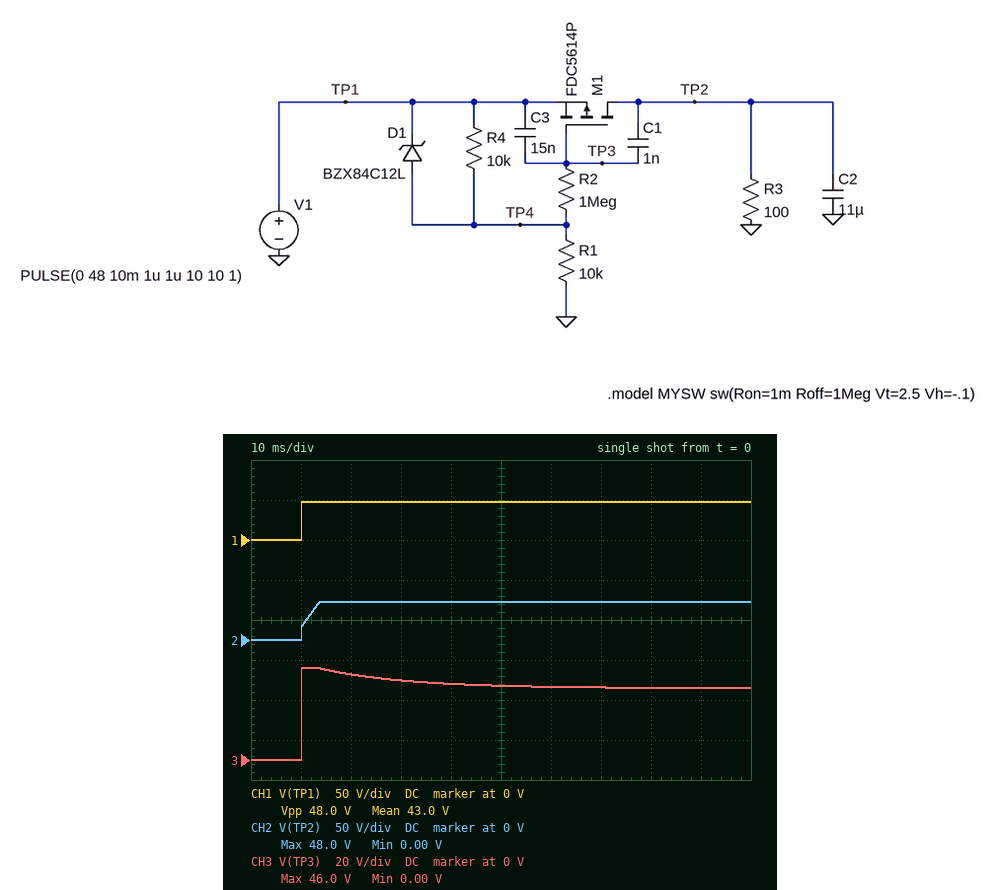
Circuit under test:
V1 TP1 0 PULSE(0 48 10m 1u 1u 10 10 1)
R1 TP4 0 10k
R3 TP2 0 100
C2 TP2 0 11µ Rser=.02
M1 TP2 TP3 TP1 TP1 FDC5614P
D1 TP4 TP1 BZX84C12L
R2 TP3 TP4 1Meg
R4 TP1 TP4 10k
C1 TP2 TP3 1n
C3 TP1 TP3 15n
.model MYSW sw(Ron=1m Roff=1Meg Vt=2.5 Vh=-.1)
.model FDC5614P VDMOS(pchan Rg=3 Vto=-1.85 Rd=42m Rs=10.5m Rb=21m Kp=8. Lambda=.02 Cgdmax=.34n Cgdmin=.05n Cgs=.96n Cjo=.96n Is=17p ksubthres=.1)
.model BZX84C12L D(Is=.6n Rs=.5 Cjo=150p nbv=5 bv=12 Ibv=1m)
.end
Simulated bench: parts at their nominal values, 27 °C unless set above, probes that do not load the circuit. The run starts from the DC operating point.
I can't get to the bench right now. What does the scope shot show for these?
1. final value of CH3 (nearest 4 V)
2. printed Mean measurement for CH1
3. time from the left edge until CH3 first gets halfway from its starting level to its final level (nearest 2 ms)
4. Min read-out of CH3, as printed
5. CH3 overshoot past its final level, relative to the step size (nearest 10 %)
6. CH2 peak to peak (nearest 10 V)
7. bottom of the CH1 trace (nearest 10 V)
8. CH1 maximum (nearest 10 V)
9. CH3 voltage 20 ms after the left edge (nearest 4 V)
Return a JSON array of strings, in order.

["36 V", "43.0 V", "10 ms", "0.00 V", "30 %", "50 V", "0 V", "50 V", "44 V"]
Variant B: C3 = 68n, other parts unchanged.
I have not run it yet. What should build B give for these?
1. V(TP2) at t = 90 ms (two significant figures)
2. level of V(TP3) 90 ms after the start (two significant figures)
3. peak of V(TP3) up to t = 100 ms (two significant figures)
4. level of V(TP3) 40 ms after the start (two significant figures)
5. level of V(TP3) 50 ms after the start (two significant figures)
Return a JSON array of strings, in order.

["48 V", "40 V", "47 V", "44 V", "43 V"]
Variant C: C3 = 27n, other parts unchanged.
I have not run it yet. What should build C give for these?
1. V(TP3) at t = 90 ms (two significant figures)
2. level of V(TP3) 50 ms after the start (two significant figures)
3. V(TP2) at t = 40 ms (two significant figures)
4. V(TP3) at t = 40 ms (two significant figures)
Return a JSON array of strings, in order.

["37 V", "39 V", "48 V", "40 V"]
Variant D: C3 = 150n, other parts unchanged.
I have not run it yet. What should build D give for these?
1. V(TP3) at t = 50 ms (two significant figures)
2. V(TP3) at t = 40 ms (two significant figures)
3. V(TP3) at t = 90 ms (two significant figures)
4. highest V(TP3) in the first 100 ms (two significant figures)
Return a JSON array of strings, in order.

["45 V", "46 V", "43 V", "48 V"]
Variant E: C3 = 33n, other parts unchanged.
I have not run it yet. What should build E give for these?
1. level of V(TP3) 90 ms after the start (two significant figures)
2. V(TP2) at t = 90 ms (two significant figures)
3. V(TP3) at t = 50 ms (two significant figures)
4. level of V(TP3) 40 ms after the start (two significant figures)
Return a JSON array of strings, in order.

["37 V", "48 V", "40 V", "41 V"]
